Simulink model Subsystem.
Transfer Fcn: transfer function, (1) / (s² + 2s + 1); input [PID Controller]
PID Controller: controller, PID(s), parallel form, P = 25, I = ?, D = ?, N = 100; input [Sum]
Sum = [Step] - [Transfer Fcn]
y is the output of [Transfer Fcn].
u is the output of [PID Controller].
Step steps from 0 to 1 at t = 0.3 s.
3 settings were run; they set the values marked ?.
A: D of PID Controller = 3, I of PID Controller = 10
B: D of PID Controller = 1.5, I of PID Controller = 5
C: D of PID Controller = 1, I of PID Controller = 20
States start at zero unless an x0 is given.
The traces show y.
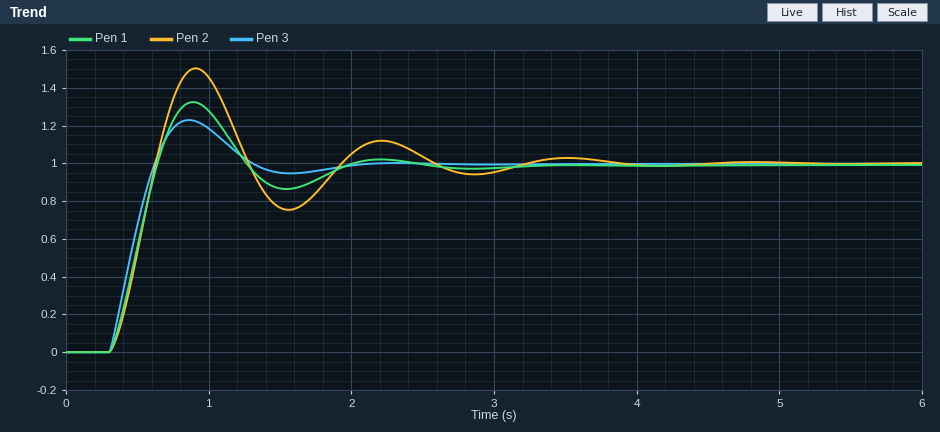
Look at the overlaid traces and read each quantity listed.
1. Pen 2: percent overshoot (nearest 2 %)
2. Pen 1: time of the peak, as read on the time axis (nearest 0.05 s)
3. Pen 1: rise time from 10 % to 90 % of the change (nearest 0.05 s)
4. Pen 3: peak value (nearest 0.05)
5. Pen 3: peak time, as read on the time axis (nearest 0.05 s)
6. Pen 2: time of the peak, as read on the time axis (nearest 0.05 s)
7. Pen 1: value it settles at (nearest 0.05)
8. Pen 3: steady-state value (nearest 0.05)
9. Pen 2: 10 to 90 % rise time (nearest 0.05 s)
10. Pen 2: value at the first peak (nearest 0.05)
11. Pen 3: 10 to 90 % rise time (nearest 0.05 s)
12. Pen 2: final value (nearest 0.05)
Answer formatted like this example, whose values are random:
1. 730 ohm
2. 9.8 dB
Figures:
1. 50 %
2. 0.90 s
3. 0.25 s
4. 1.25
5. 0.85 s
6. 0.90 s
7. 1.00
8. 1.00
9. 0.25 s
10. 1.50
11. 0.25 s
12. 1.00
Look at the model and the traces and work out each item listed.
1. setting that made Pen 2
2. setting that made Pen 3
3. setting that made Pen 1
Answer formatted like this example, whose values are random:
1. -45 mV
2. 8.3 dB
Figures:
1. C
2. A
3. B
